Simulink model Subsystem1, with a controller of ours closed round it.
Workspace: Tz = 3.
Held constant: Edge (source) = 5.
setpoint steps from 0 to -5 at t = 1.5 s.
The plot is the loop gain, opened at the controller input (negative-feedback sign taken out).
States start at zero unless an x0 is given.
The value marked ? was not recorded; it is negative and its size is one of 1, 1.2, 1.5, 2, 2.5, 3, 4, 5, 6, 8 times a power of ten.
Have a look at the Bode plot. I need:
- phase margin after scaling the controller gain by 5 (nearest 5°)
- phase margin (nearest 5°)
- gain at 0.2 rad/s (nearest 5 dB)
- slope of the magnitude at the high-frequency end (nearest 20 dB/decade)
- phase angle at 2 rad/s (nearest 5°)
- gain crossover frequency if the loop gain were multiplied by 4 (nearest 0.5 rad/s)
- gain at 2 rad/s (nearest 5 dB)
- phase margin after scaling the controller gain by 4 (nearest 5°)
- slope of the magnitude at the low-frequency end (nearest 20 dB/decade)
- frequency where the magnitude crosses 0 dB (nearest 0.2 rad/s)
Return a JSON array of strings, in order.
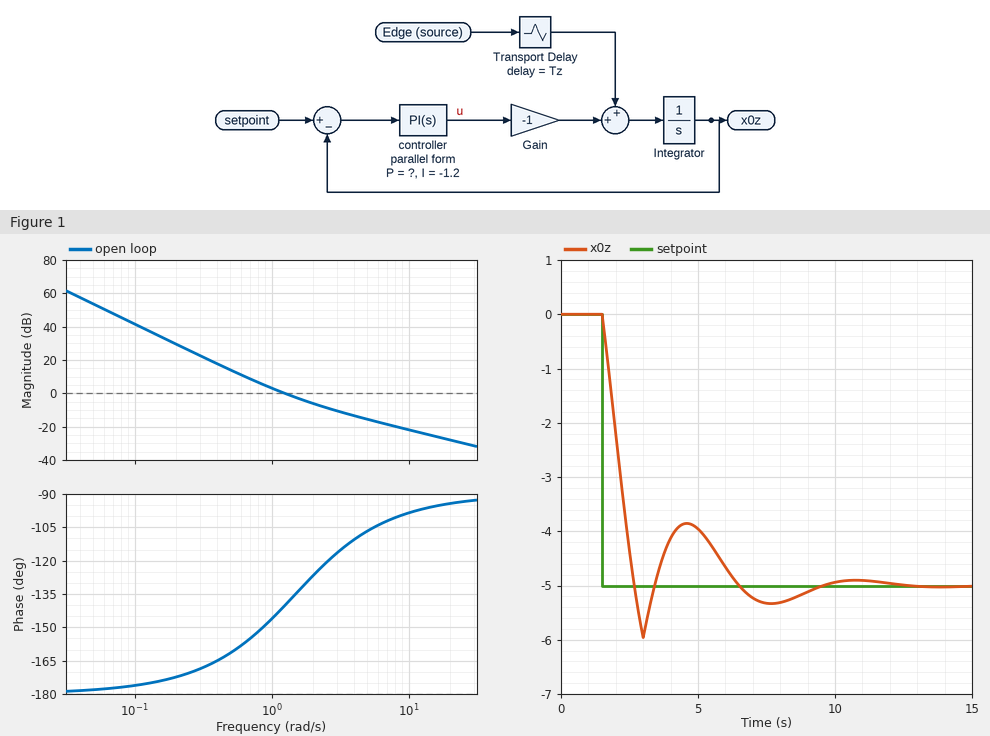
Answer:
["70°", "40°", "30 dB", "-20 dB/decade", "-125°", "3.5 rad/s", "-5 dB", "65°", "-40 dB/decade", "1.2 rad/s"]
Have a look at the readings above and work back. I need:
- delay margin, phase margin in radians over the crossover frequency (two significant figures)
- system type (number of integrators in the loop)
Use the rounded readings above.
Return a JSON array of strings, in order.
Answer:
["0.58 s", "2"]
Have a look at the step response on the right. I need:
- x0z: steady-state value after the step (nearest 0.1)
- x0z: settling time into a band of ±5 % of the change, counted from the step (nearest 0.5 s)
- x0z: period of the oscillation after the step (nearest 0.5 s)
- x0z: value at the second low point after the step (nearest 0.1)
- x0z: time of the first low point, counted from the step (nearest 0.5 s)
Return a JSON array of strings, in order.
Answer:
["-5.0", "7.0 s", "4.5 s", "-5.3", "1.5 s"]
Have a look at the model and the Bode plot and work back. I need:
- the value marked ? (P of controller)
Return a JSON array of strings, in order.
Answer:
["-0.8"]
